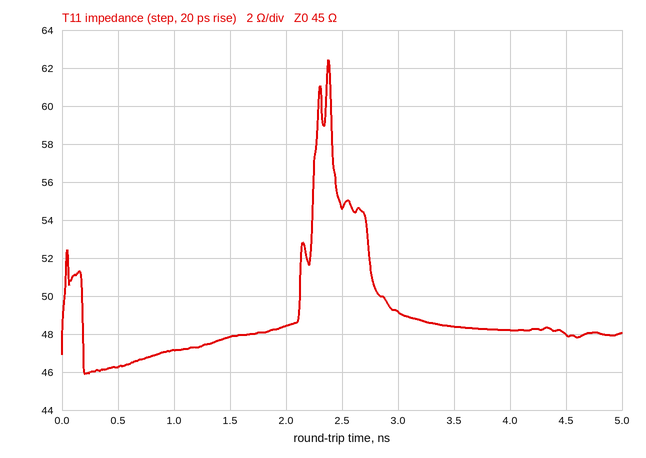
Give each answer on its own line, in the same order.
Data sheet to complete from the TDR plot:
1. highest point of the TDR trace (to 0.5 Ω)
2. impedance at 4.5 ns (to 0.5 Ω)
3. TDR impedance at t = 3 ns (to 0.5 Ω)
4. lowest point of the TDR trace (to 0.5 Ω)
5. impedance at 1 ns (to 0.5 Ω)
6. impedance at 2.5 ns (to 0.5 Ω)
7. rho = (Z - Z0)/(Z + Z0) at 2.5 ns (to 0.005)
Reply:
62.5 Ω
48.0 Ω
49.0 Ω
46.0 Ω
47.0 Ω
54.5 Ω
+0.095
